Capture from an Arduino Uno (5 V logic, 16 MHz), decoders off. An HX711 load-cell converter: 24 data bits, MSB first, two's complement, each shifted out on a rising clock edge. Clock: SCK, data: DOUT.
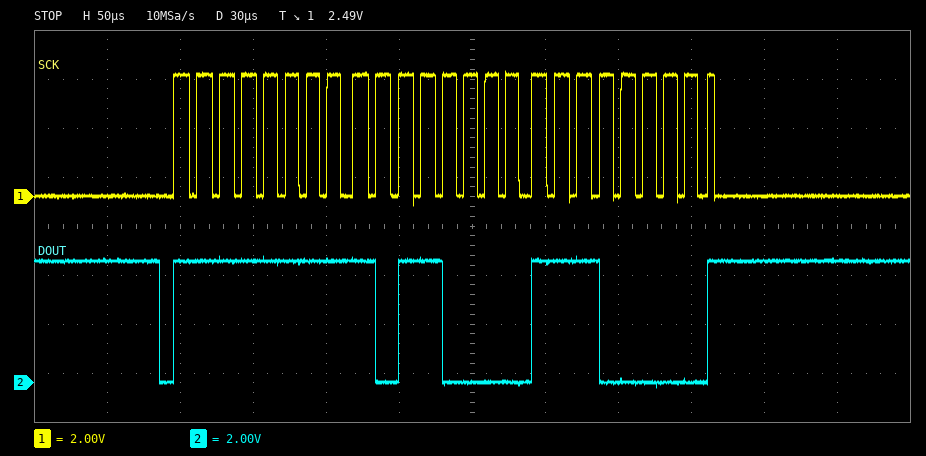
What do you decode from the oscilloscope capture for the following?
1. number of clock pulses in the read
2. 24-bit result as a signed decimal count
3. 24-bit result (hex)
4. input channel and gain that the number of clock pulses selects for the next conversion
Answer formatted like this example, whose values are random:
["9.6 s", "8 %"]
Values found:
["25", "-20256", "0xFFB0E0", "channel A, gain 128"]
